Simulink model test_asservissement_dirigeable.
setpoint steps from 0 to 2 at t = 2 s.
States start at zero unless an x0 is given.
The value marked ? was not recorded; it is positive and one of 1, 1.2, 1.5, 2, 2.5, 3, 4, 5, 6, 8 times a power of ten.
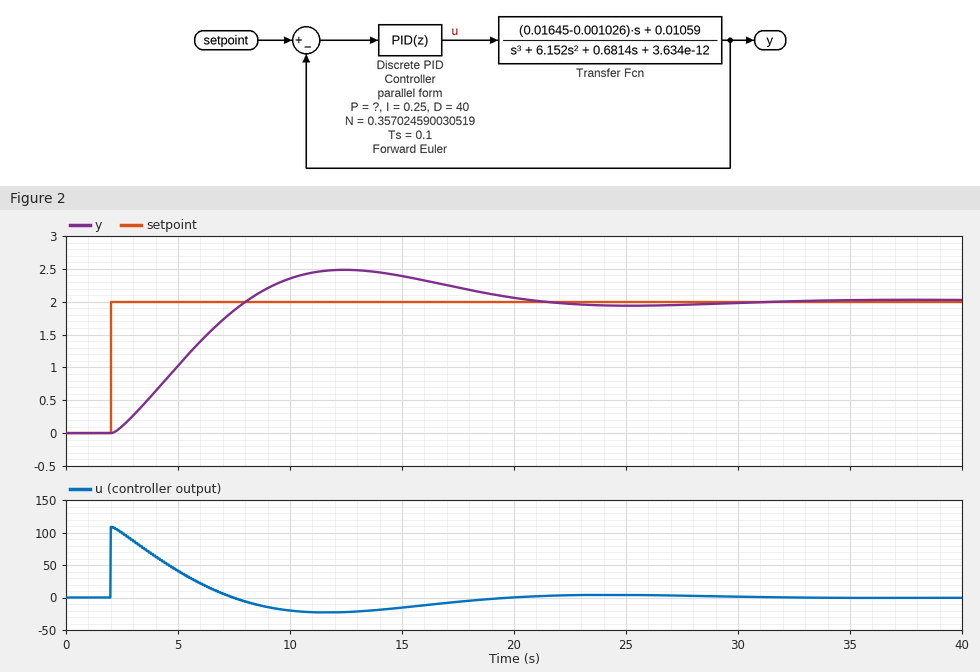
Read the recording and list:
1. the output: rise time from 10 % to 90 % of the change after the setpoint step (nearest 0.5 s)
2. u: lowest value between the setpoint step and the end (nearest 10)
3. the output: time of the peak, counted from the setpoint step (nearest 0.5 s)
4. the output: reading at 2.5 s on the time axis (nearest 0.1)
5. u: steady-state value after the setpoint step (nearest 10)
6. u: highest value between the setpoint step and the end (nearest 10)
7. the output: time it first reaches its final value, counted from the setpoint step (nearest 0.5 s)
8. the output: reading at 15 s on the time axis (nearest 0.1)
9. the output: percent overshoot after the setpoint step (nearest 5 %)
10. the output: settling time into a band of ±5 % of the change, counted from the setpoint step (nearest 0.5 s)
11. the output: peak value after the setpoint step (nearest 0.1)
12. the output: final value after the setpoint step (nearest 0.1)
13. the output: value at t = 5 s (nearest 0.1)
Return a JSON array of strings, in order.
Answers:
["4.5 s", "-20", "10.5 s", "0.1", "0", "110", "6.0 s", "2.4", "25 %", "17.0 s", "2.5", "2.0", "1.0"]
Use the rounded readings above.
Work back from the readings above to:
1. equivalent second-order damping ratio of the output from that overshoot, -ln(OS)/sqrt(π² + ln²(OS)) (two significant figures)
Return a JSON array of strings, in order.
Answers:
["0.40"]
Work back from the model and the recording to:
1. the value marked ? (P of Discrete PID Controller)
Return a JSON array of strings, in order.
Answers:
["40"]
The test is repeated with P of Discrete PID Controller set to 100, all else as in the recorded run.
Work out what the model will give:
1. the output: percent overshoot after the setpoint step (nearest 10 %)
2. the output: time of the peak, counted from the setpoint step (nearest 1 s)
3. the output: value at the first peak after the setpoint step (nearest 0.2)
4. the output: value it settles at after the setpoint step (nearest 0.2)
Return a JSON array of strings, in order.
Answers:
["30 %", "6 s", "2.6", "2.0"]
